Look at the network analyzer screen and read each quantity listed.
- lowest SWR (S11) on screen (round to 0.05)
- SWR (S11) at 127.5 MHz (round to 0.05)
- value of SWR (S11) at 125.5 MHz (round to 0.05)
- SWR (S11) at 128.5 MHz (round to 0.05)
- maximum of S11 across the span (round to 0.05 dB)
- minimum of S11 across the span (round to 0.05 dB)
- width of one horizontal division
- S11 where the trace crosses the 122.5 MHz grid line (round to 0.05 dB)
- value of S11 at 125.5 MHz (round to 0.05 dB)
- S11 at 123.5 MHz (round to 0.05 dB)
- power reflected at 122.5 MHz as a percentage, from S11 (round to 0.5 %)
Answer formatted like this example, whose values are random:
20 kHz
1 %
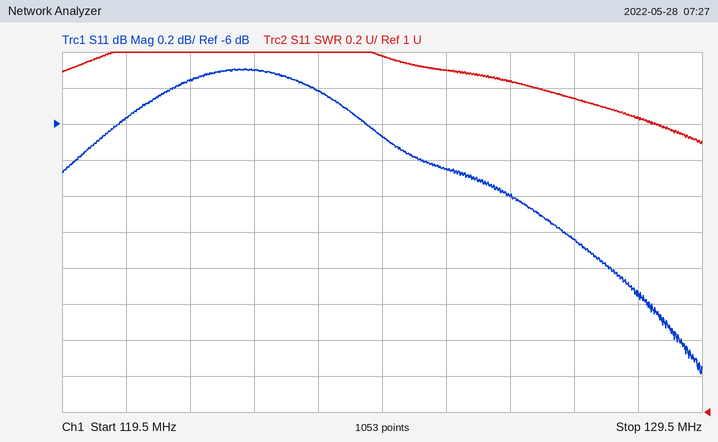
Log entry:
2.50
2.75
2.90
2.65
-5.70 dB
-7.40 dB
1 MHz
-5.70 dB
-6.25 dB
-5.80 dB
27.0 %
